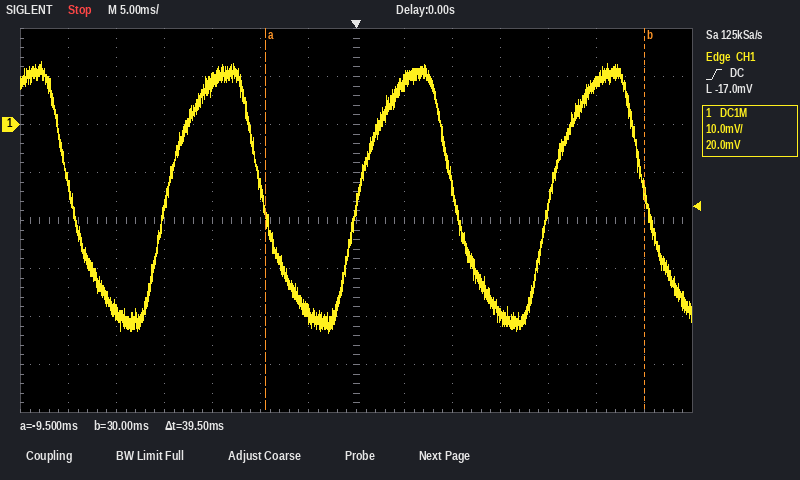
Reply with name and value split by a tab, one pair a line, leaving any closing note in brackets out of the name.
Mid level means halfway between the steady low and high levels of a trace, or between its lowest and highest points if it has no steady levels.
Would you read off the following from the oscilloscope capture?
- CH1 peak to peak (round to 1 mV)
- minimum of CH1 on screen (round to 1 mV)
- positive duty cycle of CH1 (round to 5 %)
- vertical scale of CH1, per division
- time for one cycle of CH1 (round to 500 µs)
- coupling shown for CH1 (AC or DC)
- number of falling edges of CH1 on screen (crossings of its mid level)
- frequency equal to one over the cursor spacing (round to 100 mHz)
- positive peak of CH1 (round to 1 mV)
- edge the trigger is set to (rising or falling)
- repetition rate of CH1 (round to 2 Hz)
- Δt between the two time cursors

CH1 peak to peak	57 mV
minimum of CH1 on screen	-44 mV
positive duty cycle of CH1	50 %
vertical scale of CH1, per division	10 mV
time for one cycle of CH1	20.0 ms
coupling shown for CH1	DC
number of falling edges of CH1 on screen	4
frequency equal to one over the cursor spacing	25.3 Hz
positive peak of CH1	13 mV
edge the trigger is set to	rising
repetition rate of CH1	50 Hz
Δt between the two time cursors	39.5 ms
